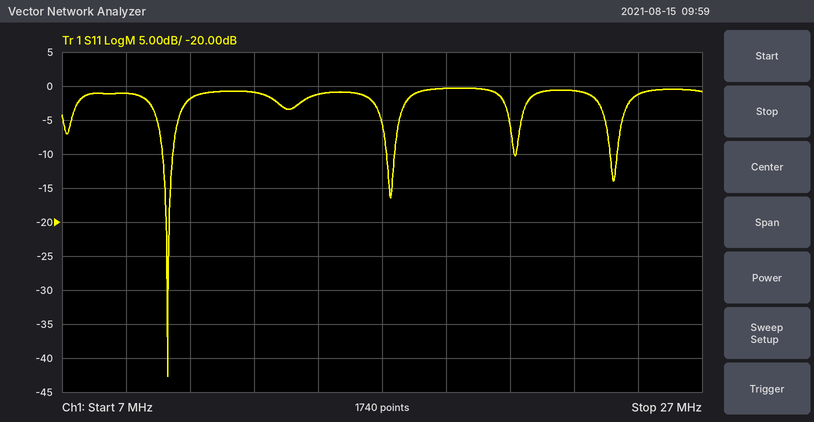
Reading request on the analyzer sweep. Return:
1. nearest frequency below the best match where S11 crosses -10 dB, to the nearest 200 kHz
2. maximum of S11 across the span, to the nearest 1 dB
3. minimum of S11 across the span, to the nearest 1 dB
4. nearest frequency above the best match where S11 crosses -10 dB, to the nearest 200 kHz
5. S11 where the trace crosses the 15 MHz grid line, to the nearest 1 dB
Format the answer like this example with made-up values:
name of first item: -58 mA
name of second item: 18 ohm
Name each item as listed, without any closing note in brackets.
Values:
nearest frequency below the best match where S11 crosses -10 dB, to the nearest 200 kHz: 10.2 MHz
maximum of S11 across the span, to the nearest 1 dB: 0 dB
minimum of S11 across the span, to the nearest 1 dB: -43 dB
nearest frequency above the best match where S11 crosses -10 dB, to the nearest 200 kHz: 10.4 MHz
S11 where the trace crosses the 15 MHz grid line, to the nearest 1 dB: -1 dB
